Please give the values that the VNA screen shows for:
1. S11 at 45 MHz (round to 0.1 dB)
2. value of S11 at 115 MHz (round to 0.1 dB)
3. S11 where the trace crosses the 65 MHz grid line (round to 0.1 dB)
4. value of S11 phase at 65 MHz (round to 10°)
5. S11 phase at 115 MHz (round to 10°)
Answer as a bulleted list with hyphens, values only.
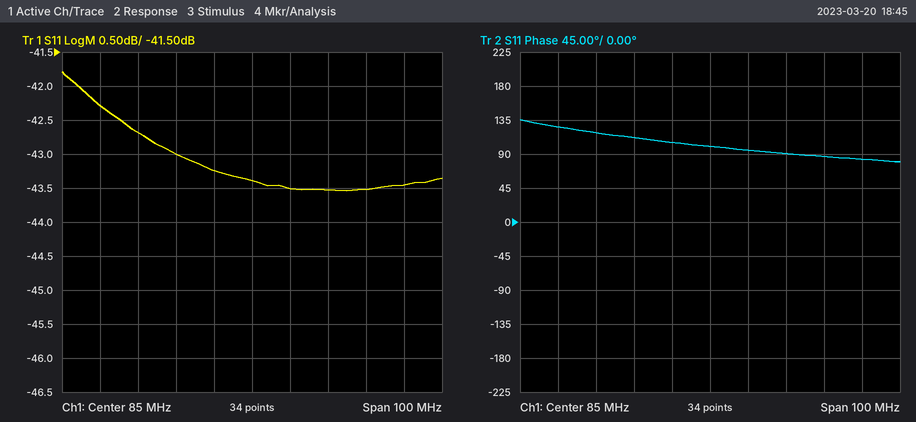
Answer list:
- -42.3 dB
- -43.5 dB
- -43.0 dB
- 110°
- 90°
